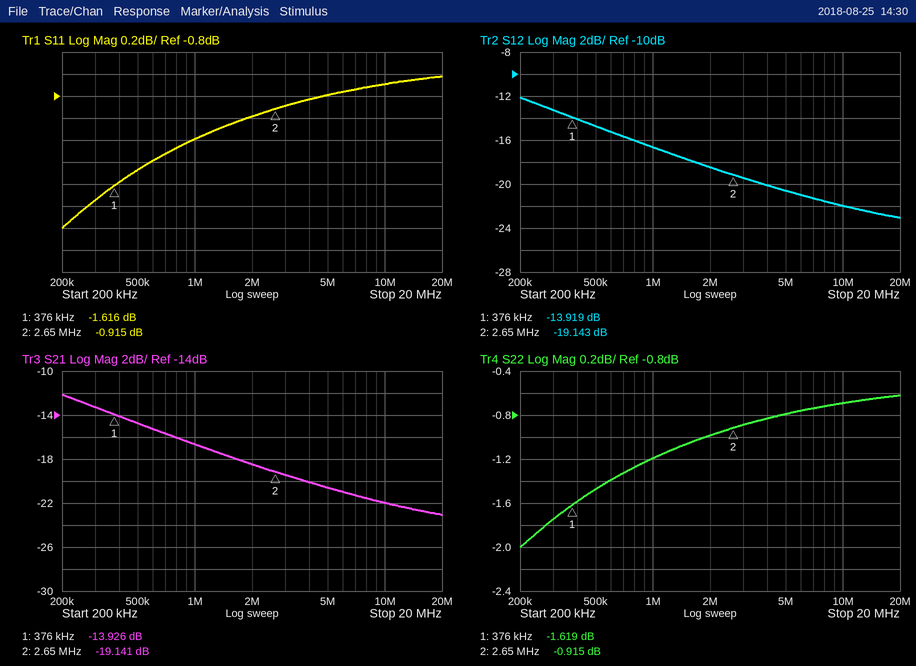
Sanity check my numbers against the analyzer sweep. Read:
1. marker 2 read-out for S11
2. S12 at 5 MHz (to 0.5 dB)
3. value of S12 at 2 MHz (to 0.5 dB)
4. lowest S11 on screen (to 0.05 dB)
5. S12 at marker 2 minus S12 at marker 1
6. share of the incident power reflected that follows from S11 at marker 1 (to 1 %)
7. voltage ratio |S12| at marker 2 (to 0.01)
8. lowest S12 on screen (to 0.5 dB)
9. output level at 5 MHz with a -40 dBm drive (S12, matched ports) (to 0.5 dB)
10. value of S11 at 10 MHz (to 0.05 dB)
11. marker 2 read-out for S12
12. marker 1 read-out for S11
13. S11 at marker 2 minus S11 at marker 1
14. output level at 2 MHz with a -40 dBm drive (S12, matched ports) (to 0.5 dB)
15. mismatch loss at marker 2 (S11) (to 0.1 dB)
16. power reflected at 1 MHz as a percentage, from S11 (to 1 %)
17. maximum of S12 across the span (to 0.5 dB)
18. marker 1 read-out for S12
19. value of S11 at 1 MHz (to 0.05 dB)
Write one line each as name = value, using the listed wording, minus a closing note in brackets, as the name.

marker 2 read-out for S11 = -0.915 dB
S12 at 5 MHz = -20.5 dB
value of S12 at 2 MHz = -18.5 dB
lowest S11 on screen = -2.00 dB
S12 at marker 2 minus S12 at marker 1 = -5.224 dB
share of the incident power reflected that follows from S11 at marker 1 = 69 %
voltage ratio |S12| at marker 2 = 0.11
lowest S12 on screen = -23.0 dB
output level at 5 MHz with a -40 dBm drive (S12, matched ports) = -60.5 dBm
value of S11 at 10 MHz = -0.70 dB
marker 2 read-out for S12 = -19.143 dB
marker 1 read-out for S11 = -1.616 dB
S11 at marker 2 minus S11 at marker 1 = 0.701 dB
output level at 2 MHz with a -40 dBm drive (S12, matched ports) = -58.5 dBm
mismatch loss at marker 2 (S11) = 7.2 dB
power reflected at 1 MHz as a percentage, from S11 = 76 %
maximum of S12 across the span = -12.0 dB
marker 1 read-out for S12 = -13.919 dB
value of S11 at 1 MHz = -1.20 dB
